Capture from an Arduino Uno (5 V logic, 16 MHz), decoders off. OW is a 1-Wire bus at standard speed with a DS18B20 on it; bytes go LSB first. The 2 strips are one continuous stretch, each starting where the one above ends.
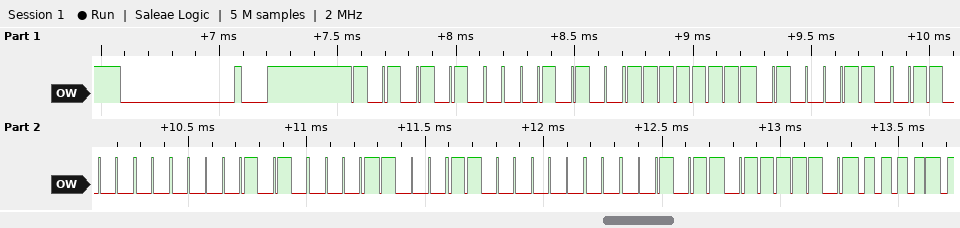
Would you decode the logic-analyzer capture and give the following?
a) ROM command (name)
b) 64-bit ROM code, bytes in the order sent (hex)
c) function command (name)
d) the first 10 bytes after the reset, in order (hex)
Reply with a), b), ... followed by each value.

a) Match ROM
b) 28 FF 62 06 50 18 03 D0
c) Read Scratchpad
d) 55 28 FF 62 06 50 18 03 D0 BE
